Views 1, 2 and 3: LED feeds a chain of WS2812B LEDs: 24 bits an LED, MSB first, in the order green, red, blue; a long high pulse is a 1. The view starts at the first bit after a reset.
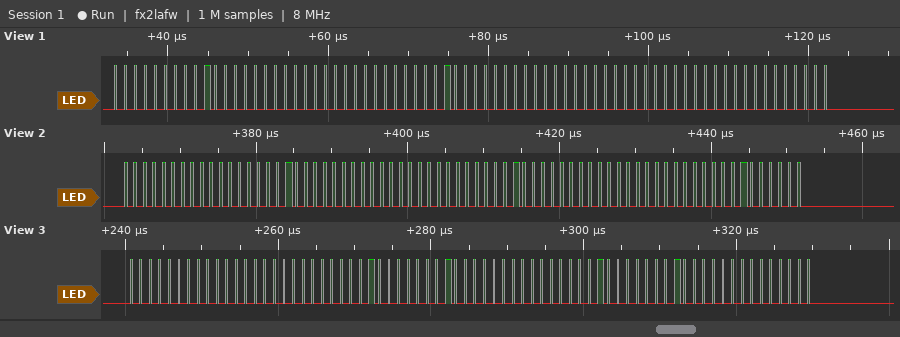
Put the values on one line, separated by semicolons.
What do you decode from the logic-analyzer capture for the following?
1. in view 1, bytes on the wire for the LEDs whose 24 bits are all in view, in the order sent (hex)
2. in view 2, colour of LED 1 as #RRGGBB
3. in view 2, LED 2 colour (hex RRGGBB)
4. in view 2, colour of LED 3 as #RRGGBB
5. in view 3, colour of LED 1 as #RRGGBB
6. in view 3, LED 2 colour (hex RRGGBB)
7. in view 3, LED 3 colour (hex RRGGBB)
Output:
00 40 00 00 40 00 00 00 00; #000040; #000040; #000040; #000000; #404000; #404000
